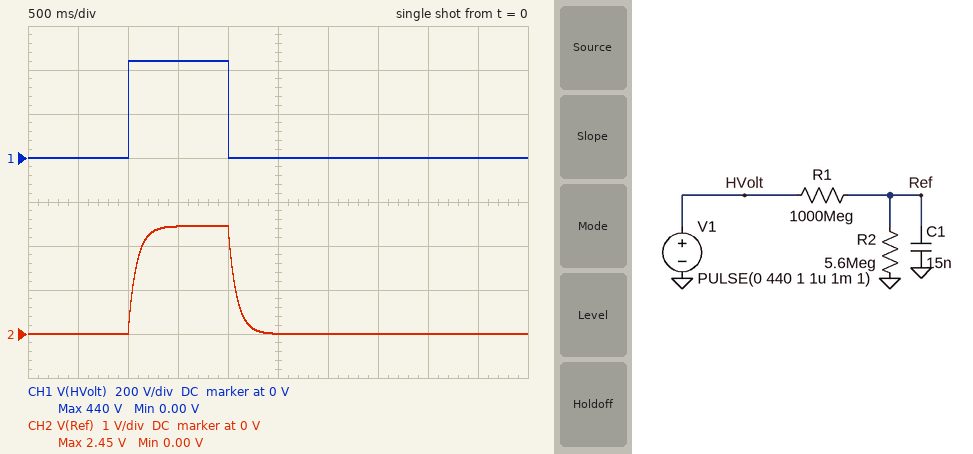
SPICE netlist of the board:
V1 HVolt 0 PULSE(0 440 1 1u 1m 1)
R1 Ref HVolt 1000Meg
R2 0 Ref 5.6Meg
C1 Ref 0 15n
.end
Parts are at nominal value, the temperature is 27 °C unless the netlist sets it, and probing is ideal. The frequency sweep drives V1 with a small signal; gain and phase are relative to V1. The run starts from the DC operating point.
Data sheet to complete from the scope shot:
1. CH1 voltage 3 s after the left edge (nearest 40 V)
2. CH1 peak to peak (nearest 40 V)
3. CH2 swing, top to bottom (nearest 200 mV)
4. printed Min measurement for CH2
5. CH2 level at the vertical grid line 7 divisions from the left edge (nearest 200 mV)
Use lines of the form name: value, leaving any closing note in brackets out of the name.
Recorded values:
CH1 voltage 3 s after the left edge: 0 V
CH1 peak to peak: 440 V
CH2 swing, top to bottom: 2.4 V
printed Min measurement for CH2: 0.00 V
CH2 level at the vertical grid line 7 divisions from the left edge: 0 V
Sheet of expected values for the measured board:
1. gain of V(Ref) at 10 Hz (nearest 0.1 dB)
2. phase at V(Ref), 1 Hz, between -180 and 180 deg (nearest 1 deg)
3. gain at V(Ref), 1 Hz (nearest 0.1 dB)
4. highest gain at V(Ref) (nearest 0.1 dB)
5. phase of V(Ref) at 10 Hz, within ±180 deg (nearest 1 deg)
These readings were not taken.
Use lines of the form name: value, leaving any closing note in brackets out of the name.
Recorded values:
gain of V(Ref) at 10 Hz: -59.6 dB
phase at V(Ref), 1 Hz, between -180 and 180 deg: -28 deg
gain at V(Ref), 1 Hz: -46.1 dB
highest gain at V(Ref): -45.1 dB
phase of V(Ref) at 10 Hz, within ±180 deg: -79 deg
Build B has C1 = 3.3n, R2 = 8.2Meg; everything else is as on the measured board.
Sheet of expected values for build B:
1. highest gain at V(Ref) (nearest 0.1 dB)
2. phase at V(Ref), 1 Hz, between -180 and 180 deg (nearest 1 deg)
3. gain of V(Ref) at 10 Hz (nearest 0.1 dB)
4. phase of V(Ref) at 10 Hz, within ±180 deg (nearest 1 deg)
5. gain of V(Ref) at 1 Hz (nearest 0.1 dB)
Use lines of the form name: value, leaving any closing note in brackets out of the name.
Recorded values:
highest gain at V(Ref): -41.8 dB
phase at V(Ref), 1 Hz, between -180 and 180 deg: -10 deg
gain of V(Ref) at 10 Hz: -47.6 dB
phase of V(Ref) at 10 Hz, within ±180 deg: -59 deg
gain of V(Ref) at 1 Hz: -41.9 dB
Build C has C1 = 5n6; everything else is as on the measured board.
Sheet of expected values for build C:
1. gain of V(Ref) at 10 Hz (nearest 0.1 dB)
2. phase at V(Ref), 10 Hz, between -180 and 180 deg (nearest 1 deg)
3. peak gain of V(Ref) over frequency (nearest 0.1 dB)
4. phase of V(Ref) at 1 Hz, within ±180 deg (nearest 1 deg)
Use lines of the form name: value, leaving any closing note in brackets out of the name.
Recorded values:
gain of V(Ref) at 10 Hz: -51.9 dB
phase at V(Ref), 10 Hz, between -180 and 180 deg: -63 deg
peak gain of V(Ref) over frequency: -45.1 dB
phase of V(Ref) at 1 Hz, within ±180 deg: -11 deg
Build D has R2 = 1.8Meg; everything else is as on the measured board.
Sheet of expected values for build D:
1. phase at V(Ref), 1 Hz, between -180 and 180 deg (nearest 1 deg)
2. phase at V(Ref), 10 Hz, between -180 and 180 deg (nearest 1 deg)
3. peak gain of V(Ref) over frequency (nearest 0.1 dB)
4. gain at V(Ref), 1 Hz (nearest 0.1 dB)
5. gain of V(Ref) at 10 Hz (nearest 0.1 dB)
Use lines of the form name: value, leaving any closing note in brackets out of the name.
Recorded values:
phase at V(Ref), 1 Hz, between -180 and 180 deg: -10 deg
phase at V(Ref), 10 Hz, between -180 and 180 deg: -59 deg
peak gain of V(Ref) over frequency: -54.9 dB
gain at V(Ref), 1 Hz: -55.0 dB
gain of V(Ref) at 10 Hz: -60.8 dB
